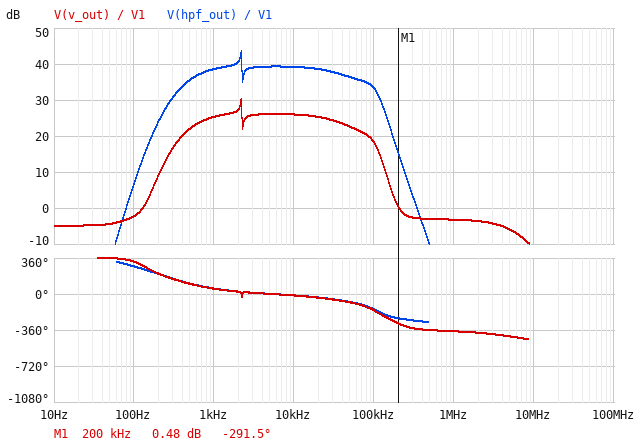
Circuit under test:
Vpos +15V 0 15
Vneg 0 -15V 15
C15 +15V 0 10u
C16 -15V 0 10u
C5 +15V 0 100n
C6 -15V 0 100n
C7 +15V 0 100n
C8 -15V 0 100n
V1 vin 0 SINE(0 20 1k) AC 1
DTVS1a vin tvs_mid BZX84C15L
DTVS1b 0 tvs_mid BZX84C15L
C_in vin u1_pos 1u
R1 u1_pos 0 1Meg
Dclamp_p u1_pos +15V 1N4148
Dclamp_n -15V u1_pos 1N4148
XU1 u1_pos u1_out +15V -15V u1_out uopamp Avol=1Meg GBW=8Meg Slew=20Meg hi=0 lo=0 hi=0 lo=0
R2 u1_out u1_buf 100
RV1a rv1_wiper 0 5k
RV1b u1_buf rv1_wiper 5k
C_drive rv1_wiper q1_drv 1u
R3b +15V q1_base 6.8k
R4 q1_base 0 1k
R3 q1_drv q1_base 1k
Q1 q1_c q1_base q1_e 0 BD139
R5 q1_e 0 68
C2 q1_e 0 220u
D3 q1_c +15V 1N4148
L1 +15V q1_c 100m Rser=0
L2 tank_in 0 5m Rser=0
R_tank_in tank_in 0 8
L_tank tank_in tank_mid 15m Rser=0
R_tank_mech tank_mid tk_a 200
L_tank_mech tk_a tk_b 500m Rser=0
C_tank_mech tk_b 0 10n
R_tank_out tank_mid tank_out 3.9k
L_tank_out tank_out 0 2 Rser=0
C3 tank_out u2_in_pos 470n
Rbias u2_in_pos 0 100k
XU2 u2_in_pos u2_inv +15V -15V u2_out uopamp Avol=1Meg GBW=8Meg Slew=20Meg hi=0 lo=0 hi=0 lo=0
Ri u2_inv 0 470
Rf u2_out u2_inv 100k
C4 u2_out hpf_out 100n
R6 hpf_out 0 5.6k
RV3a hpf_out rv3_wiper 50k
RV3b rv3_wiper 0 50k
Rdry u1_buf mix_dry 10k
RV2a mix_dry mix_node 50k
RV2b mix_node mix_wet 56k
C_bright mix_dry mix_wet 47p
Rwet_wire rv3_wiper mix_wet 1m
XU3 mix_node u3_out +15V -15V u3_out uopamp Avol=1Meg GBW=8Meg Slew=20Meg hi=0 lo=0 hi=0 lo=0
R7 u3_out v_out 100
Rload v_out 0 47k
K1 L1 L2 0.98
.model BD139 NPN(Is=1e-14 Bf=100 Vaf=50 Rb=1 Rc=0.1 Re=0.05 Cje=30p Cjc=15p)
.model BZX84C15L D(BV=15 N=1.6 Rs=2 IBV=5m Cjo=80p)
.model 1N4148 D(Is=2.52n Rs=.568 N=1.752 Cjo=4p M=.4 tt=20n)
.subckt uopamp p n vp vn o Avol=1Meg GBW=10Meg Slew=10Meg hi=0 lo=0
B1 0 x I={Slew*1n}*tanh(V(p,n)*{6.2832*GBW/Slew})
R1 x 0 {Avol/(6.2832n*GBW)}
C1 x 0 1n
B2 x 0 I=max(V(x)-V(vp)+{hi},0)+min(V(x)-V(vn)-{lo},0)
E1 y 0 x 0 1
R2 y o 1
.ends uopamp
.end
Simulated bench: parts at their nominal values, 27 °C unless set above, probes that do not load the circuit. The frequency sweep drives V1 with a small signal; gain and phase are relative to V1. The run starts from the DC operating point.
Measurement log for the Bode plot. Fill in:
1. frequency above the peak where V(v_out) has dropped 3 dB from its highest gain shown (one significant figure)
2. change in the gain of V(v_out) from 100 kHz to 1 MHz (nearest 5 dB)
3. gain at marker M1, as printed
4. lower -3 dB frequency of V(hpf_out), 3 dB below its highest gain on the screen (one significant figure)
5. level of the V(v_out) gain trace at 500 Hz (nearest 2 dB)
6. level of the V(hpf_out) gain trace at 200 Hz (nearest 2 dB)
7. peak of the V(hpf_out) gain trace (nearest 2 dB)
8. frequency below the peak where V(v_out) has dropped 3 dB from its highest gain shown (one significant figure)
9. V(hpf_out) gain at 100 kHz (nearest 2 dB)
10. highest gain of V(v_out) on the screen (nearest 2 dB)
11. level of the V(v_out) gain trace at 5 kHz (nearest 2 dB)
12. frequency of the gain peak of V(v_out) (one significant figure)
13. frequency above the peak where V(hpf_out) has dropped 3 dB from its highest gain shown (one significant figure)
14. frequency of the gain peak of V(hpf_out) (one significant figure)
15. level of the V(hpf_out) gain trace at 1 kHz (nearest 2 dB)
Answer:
2 kHz
-20 dB
0.48 dB
2 kHz
22 dB
24 dB
44 dB
2 kHz
34 dB
30 dB
26 dB
2 kHz
2 kHz
2 kHz
38 dB
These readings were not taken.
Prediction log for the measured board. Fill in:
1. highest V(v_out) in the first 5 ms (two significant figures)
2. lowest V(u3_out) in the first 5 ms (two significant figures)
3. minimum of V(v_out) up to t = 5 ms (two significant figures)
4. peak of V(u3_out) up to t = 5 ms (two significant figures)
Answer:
14 V
-12 V
-12 V
14 V
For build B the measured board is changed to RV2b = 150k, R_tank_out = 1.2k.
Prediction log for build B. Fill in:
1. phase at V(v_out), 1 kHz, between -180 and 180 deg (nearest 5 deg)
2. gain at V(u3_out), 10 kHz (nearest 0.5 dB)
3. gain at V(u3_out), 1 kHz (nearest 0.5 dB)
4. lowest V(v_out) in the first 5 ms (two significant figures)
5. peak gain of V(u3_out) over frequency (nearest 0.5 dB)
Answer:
40 deg
22.0 dB
21.5 dB
-13 V
26.5 dB
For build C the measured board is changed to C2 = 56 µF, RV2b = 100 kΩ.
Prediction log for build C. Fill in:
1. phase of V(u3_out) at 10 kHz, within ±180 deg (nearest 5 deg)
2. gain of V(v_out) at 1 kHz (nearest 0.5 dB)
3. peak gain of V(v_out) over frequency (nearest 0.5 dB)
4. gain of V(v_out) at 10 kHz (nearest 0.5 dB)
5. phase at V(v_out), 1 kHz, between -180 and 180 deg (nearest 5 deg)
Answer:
-10 deg
22.0 dB
28.0 dB
23.5 dB
65 deg
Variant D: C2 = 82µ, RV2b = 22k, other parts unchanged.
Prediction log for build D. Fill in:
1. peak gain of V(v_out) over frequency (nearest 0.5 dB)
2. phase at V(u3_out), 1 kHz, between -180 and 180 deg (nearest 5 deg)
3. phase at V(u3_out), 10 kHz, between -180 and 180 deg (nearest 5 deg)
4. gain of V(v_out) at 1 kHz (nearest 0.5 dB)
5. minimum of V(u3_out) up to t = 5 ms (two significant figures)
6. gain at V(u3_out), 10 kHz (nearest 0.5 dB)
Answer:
33.0 dB
65 deg
-15 deg
27.5 dB
-11 V
28.5 dB
